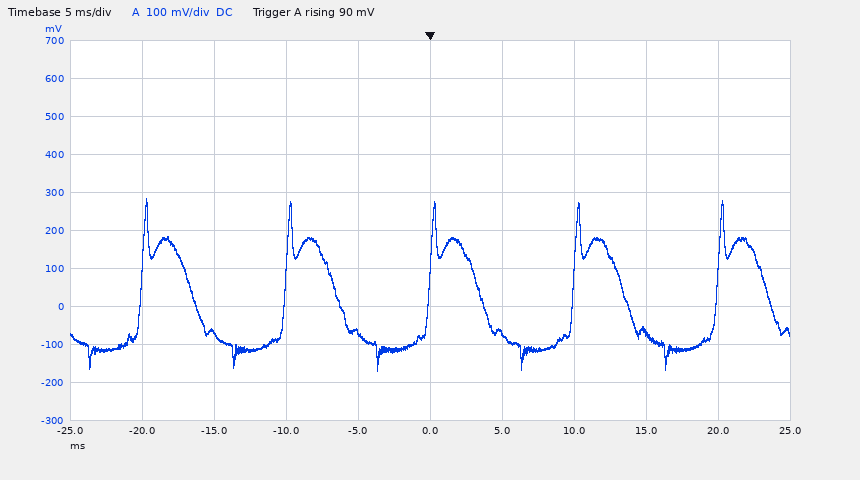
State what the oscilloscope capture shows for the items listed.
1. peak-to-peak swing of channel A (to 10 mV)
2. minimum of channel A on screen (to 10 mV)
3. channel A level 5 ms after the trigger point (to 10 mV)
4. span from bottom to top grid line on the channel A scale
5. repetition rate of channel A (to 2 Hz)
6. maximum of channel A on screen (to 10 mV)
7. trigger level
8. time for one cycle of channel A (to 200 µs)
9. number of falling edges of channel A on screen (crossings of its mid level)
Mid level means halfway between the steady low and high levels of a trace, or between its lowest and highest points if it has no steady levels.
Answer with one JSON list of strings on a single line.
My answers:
["450 mV", "-170 mV", "-70 mV", "1 V", "100 Hz", "280 mV", "90 mV", "10.0 ms", "5"]
